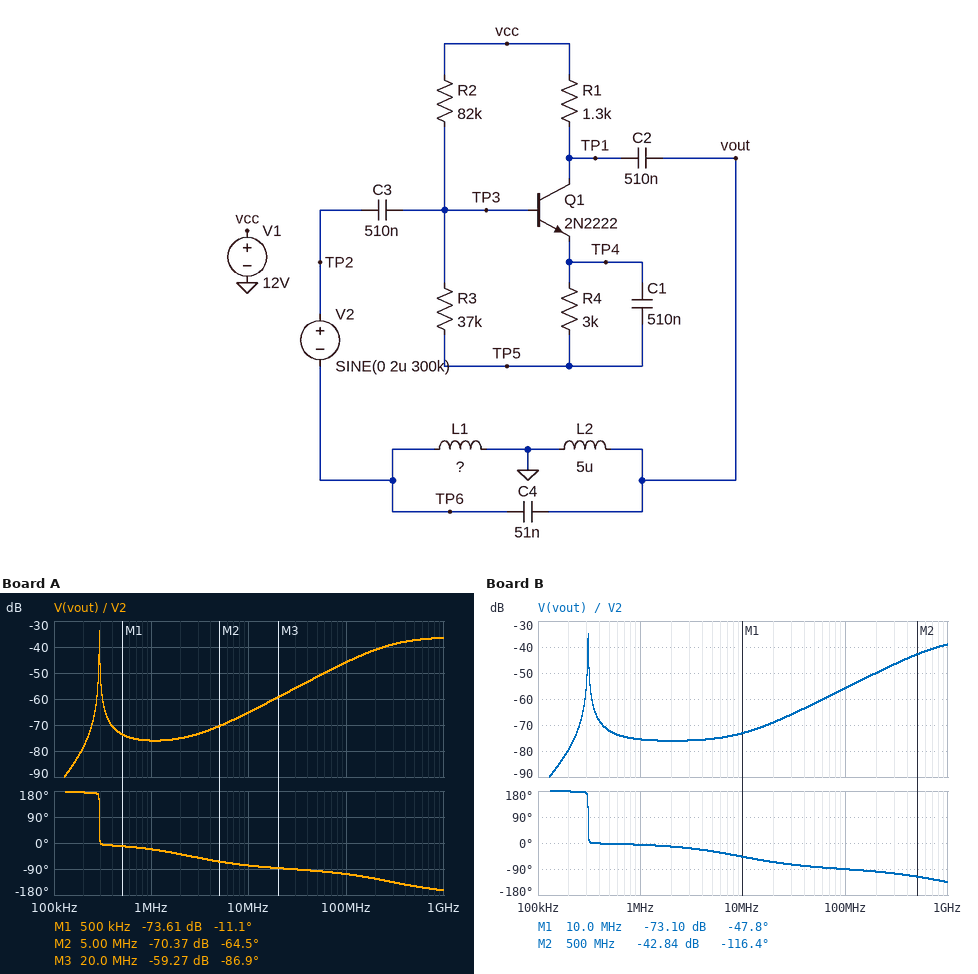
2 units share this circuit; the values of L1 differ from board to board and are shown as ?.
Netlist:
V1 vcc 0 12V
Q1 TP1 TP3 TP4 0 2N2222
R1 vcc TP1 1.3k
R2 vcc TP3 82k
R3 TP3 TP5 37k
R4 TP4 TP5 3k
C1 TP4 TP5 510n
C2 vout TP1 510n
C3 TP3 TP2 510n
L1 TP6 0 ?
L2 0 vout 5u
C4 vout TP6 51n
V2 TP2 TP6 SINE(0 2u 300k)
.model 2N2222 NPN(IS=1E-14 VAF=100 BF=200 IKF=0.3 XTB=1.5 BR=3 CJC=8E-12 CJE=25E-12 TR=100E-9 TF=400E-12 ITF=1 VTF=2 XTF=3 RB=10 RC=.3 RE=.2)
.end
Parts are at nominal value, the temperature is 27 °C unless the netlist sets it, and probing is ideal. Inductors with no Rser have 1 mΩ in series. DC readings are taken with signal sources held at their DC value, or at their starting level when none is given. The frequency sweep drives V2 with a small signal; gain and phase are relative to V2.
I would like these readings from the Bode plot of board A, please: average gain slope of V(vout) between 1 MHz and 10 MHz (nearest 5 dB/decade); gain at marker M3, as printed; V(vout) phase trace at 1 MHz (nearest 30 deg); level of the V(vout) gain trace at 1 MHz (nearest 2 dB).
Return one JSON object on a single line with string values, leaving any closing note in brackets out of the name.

{"average gain slope of V(vout) between 1 MHz and 10 MHz": "10 dB/decade", "gain at marker M3, as printed": "-59.27 dB", "V(vout) phase trace at 1 MHz": "-30 deg", "level of the V(vout) gain trace at 1 MHz": "-76 dB"}
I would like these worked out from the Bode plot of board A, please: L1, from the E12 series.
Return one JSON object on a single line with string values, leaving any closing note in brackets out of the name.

{"L1, from the E12 series": "820 nH"}
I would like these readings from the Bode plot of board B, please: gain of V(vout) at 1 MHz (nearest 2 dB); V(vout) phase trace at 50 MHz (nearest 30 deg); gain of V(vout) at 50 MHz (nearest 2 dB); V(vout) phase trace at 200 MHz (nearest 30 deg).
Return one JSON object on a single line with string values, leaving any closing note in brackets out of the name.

{"gain of V(vout) at 1 MHz": "-76 dB", "V(vout) phase trace at 50 MHz": "-90 deg", "gain of V(vout) at 50 MHz": "-62 dB", "V(vout) phase trace at 200 MHz": "-90 deg"}
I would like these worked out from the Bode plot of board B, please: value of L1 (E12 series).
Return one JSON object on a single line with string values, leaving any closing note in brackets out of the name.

{"value of L1": "220 nH"}
